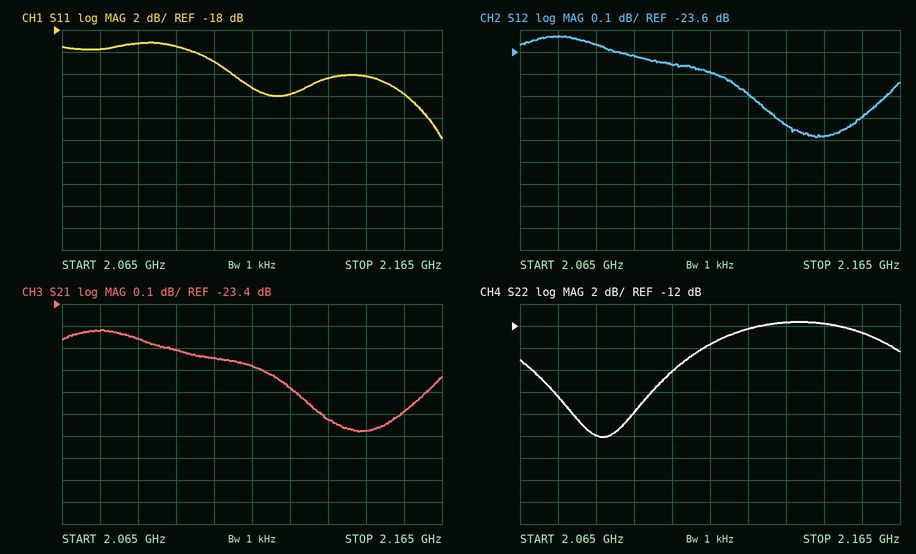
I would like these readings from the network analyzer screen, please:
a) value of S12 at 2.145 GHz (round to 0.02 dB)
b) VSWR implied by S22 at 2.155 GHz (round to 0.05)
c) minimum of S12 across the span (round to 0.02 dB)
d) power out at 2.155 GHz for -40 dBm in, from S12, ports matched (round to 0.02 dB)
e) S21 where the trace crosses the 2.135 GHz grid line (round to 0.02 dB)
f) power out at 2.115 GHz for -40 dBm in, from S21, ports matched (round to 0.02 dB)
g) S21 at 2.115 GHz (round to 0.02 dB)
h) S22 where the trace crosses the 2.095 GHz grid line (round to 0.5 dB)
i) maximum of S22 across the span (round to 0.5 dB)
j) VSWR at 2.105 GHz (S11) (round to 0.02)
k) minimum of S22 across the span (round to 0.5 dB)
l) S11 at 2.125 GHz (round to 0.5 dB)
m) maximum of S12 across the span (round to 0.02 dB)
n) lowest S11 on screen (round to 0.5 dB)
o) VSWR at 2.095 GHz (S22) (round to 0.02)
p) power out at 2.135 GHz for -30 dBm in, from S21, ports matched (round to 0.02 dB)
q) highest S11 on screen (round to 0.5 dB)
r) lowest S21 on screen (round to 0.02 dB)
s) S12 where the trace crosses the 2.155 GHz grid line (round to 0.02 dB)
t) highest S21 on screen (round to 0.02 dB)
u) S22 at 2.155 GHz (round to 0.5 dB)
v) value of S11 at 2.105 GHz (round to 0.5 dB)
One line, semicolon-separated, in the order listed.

-23.98 dB; 1.60; -23.98 dB; -63.90 dBm; -23.92 dB; -63.68 dBm; -23.68 dB; -20.0 dB; -11.5 dB; 1.20; -22.0 dB; -24.0 dB; -23.52 dB; -28.0 dB; 1.22; -53.92 dBm; -19.0 dB; -23.98 dB; -23.90 dB; -23.52 dB; -12.5 dB; -21.0 dB
